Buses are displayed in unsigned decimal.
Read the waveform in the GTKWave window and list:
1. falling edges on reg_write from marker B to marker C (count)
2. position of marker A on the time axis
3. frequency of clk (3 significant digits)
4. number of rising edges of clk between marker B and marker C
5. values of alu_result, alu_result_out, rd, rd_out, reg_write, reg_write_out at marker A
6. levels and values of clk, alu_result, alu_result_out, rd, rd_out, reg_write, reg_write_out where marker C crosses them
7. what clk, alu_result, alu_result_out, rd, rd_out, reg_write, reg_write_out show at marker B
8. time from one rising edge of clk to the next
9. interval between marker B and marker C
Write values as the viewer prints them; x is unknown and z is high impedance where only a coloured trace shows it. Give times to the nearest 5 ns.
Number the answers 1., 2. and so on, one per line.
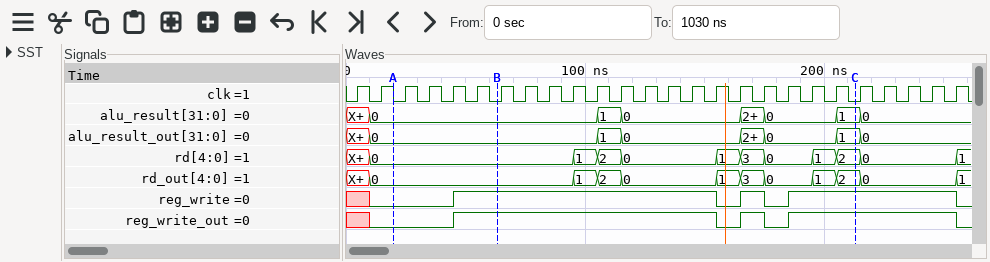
1. 2
2. 20 ns
3. 100 MHz
4. 15
5. alu_result=0, alu_result_out=0, rd=0, rd_out=0, reg_write=0, reg_write_out=0
6. clk=0, alu_result=1, alu_result_out=1, rd=2, rd_out=2, reg_write=1, reg_write_out=1
7. clk=0, alu_result=0, alu_result_out=0, rd=0, rd_out=0, reg_write=1, reg_write_out=1
8. 10 ns
9. 150 ns
